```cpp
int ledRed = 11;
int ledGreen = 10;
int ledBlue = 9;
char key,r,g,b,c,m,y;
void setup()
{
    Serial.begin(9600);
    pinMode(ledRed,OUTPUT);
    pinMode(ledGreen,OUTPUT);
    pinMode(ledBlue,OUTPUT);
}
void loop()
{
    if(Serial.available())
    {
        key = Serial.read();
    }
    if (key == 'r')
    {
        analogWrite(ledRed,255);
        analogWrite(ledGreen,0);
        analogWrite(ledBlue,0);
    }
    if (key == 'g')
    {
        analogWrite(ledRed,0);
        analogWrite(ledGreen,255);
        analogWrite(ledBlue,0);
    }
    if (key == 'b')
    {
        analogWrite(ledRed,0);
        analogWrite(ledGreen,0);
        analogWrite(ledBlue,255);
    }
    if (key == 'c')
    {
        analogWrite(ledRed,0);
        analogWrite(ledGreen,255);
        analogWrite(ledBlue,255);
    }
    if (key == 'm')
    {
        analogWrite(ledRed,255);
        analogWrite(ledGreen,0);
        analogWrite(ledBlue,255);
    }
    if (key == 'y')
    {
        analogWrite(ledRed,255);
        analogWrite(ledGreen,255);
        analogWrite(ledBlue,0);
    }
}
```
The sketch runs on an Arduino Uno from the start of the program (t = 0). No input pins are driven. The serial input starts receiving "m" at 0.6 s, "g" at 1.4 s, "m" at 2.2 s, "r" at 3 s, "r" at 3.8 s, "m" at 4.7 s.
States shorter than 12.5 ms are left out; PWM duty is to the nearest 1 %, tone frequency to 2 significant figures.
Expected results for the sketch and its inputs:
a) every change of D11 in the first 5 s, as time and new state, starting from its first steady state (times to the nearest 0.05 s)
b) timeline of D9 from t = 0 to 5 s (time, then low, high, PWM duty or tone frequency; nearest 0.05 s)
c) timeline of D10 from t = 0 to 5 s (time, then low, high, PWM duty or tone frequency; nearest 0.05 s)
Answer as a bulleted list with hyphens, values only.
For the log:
- 0 s low; 0.6 s high; 1.4 s low; 2.2 s high
- 0 s low; 0.6 s high; 1.4 s low; 2.2 s high; 3 s low; 4.7 s high
- 0 s low; 1.4 s high; 2.2 s low
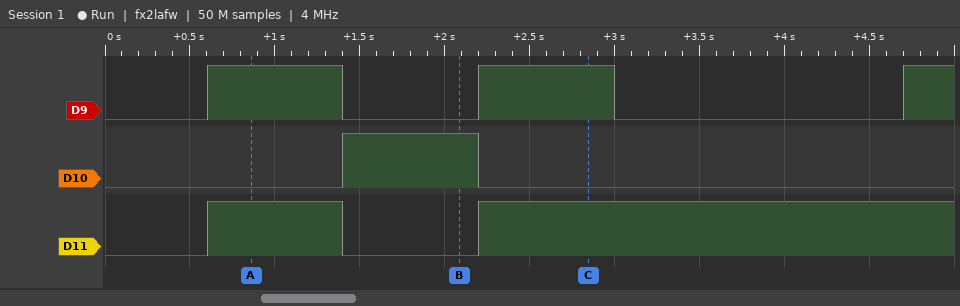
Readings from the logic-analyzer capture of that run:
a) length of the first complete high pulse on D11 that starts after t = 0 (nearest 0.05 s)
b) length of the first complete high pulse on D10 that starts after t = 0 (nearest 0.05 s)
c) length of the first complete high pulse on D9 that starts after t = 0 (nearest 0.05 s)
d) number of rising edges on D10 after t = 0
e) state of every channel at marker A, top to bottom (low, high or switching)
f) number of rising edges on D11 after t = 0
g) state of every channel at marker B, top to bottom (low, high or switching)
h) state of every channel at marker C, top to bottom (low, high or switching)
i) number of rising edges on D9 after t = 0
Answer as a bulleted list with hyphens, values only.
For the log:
- 0.80 s
- 0.80 s
- 0.80 s
- 1
- D9 high, D10 low, D11 high
- 2
- D9 low, D10 high, D11 low
- D9 high, D10 low, D11 high
- 3
